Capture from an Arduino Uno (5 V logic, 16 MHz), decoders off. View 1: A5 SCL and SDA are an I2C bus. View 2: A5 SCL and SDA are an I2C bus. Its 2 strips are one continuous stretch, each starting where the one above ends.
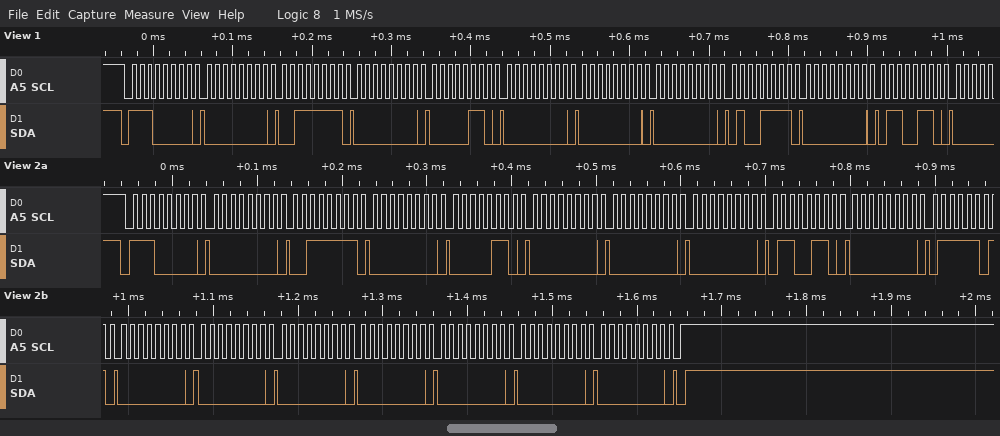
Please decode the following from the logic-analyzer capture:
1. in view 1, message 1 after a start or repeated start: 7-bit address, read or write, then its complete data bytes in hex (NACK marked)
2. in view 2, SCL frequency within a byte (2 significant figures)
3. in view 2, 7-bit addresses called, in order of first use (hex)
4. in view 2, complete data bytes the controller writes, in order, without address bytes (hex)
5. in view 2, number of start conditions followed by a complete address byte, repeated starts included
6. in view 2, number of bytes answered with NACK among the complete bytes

0x70 write: 00 3F 00 06 00 00 00 4F 00 66
100 kHz
0x70
00 3F 00 06 00 00 00 66 00 7D 00 00 00 00 00 00 00
1
0
